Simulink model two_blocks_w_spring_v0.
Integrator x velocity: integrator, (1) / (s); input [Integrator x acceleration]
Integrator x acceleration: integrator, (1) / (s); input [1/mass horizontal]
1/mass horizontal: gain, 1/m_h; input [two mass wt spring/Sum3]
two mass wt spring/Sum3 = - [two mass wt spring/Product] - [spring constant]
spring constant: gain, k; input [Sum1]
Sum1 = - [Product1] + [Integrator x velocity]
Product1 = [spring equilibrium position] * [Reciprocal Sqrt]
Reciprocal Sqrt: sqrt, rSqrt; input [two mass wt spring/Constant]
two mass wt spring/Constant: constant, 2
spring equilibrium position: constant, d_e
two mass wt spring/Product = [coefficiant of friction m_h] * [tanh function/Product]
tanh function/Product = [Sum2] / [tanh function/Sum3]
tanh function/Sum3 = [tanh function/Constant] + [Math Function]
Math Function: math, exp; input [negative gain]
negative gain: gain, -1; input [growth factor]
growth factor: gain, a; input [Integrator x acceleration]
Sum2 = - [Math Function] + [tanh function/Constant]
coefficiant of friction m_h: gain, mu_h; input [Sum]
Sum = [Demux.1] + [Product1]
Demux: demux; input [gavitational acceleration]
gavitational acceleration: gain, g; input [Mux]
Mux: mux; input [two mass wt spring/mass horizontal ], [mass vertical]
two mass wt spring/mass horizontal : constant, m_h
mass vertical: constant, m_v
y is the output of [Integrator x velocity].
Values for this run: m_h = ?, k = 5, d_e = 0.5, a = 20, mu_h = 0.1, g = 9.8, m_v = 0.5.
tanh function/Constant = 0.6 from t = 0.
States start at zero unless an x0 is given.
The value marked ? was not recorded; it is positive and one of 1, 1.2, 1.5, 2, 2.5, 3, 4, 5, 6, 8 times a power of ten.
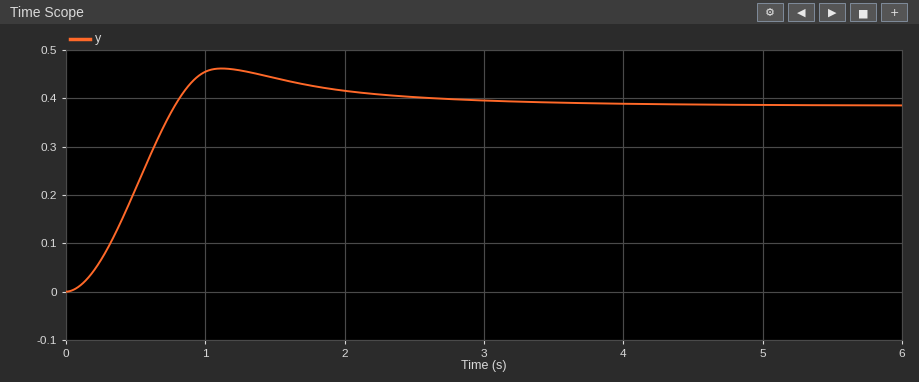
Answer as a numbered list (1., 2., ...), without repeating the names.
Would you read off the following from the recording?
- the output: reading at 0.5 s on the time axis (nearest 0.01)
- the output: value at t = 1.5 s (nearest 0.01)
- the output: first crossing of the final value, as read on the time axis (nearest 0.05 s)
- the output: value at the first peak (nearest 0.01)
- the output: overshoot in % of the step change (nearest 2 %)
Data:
1. 0.21
2. 0.44
3. 0.80 s
4. 0.46
5. 20 %
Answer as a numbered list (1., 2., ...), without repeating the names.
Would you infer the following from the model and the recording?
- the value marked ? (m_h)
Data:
1. 0.6
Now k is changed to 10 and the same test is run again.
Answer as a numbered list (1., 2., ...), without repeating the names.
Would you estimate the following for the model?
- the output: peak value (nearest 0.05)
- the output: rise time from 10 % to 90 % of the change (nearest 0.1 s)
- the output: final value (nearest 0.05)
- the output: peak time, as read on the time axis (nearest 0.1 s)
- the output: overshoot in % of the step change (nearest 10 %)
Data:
1. 0.60
2. 0.3 s
3. 0.35
4. 0.8 s
5. 60 %
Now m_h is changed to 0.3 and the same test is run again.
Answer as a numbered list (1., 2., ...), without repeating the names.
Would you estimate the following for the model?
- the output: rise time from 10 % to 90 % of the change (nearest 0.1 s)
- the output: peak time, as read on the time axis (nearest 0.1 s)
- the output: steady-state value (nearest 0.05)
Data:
1. 0.3 s
2. 0.8 s
3. 0.35
